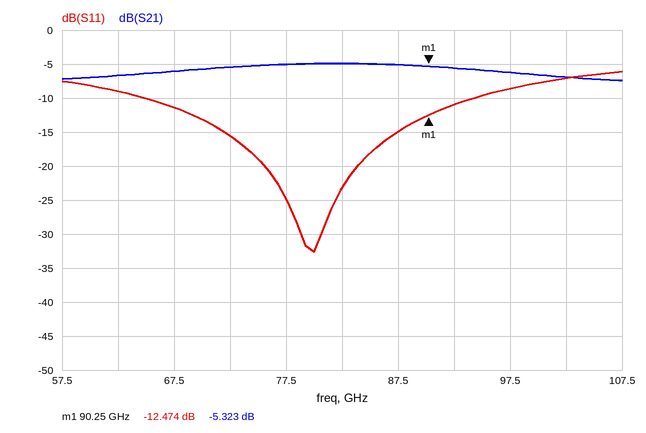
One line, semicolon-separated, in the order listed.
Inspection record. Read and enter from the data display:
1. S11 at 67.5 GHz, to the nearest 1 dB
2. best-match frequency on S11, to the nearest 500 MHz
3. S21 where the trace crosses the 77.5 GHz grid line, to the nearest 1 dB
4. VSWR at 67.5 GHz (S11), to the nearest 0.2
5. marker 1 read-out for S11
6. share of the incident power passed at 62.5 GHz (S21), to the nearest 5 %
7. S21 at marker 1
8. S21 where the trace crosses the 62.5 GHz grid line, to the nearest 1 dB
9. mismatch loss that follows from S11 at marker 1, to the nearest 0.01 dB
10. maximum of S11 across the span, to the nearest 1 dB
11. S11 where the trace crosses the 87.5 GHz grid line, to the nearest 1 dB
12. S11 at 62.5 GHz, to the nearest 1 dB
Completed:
-11 dB; 80.0 GHz; -5 dB; 1.8; -12.474 dB; 20 %; -5.323 dB; -7 dB; 0.25 dB; -6 dB; -15 dB; -9 dB
